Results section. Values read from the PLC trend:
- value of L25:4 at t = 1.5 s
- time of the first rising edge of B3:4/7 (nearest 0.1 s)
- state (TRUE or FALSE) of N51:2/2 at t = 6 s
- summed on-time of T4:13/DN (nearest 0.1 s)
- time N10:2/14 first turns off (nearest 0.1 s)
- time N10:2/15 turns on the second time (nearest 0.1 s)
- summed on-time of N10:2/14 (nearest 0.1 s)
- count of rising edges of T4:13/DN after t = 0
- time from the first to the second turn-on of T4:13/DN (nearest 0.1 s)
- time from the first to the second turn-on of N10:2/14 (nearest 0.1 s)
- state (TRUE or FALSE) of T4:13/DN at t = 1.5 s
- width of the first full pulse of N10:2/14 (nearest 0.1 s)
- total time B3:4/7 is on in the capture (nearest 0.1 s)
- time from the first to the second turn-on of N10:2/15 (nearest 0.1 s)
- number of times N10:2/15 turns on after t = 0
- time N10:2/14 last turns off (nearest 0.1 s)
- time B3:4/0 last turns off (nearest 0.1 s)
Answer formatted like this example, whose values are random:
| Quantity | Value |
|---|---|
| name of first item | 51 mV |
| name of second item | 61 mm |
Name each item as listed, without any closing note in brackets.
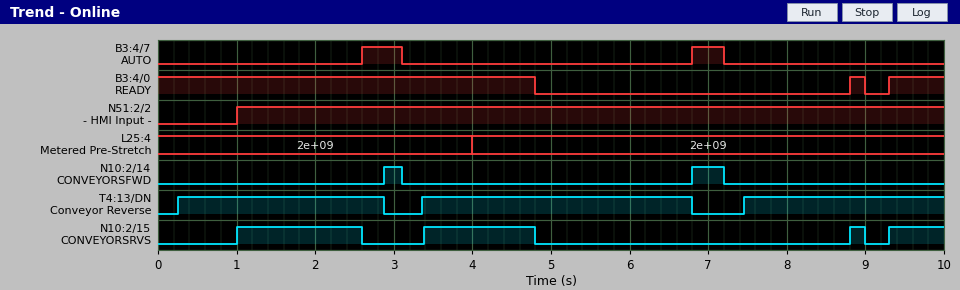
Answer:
| Quantity | Value |
|---|---|
| value of L25:4 at t = 1.5 s | 2e+09 |
| time of the first rising edge of B3:4/7 | 2.6 s |
| state (TRUE or FALSE) of N51:2/2 at t = 6 s | TRUE |
| summed on-time of T4:13/DN | 8.6 s |
| time N10:2/14 first turns off | 3.1 s |
| time N10:2/15 turns on the second time | 3.4 s |
| summed on-time of N10:2/14 | 0.6 s |
| count of rising edges of T4:13/DN after t = 0 | 3 |
| time from the first to the second turn-on of T4:13/DN | 3.1 s |
| time from the first to the second turn-on of N10:2/14 | 3.9 s |
| state (TRUE or FALSE) of T4:13/DN at t = 1.5 s | TRUE |
| width of the first full pulse of N10:2/14 | 0.2 s |
| total time B3:4/7 is on in the capture | 0.9 s |
| time from the first to the second turn-on of N10:2/15 | 2.4 s |
| number of times N10:2/15 turns on after t = 0 | 4 |
| time N10:2/14 last turns off | 7.2 s |
| time B3:4/0 last turns off | 9.0 s |
